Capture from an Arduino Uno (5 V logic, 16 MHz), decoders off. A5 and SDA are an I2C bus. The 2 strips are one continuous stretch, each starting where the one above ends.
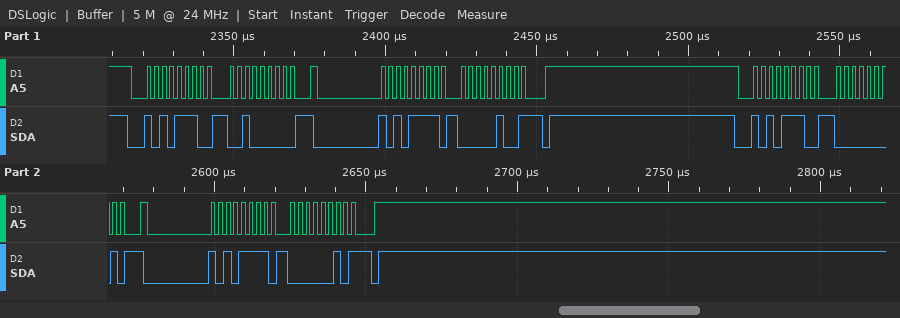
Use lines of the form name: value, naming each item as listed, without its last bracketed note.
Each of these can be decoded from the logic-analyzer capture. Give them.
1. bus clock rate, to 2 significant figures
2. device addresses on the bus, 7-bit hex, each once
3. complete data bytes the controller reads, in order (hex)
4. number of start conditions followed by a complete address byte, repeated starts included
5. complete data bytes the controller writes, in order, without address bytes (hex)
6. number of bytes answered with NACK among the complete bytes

bus clock rate, to 2 significant figures: 400 kHz
device addresses on the bus, 7-bit hex, each once: 0x57
complete data bytes the controller reads, in order: 04 02
number of start conditions followed by a complete address byte, repeated starts included: 4
complete data bytes the controller writes, in order, without address bytes: 20 01
number of bytes answered with NACK among the complete bytes: 2
